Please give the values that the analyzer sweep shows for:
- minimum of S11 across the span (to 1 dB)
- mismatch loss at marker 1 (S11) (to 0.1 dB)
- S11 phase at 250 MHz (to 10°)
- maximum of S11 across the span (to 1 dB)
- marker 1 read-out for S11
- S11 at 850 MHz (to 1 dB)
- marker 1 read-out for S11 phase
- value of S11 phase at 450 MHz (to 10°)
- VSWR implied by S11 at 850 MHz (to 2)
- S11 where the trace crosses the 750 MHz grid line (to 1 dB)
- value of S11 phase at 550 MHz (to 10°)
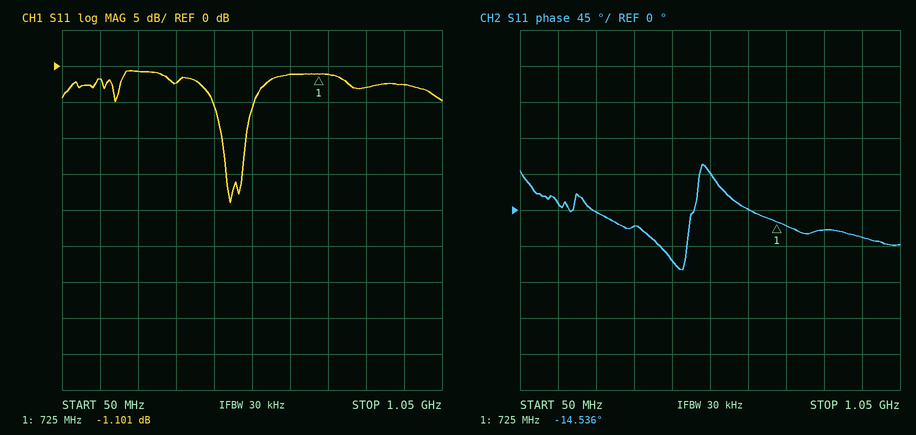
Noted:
-19 dB
6.5 dB
0°
-1 dB
-1.101 dB
-3 dB
-14.536°
-60°
6
-1 dB
50°
